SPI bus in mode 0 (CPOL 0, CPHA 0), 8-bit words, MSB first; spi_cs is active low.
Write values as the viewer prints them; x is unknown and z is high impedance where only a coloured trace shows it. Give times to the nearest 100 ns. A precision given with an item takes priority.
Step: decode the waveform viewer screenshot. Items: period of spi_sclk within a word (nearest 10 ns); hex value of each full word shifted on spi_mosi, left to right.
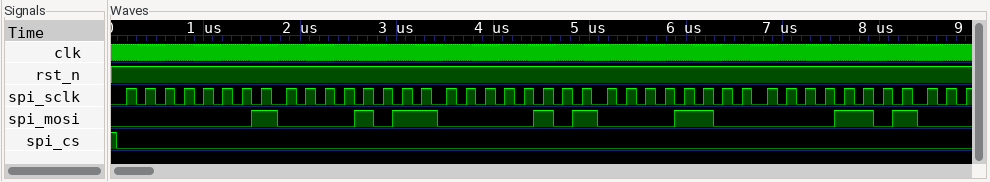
200 ns
01, 0B, 05, 0C, 0D
